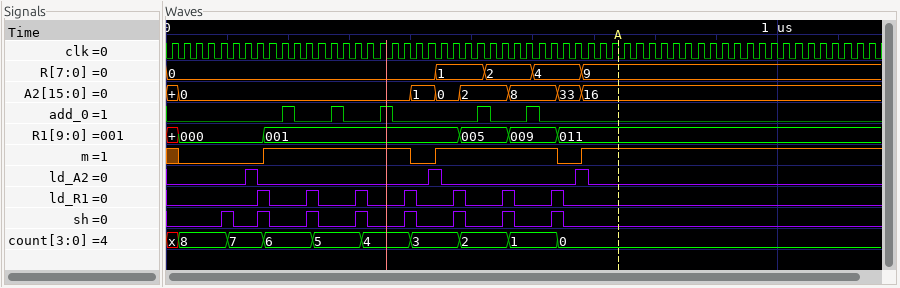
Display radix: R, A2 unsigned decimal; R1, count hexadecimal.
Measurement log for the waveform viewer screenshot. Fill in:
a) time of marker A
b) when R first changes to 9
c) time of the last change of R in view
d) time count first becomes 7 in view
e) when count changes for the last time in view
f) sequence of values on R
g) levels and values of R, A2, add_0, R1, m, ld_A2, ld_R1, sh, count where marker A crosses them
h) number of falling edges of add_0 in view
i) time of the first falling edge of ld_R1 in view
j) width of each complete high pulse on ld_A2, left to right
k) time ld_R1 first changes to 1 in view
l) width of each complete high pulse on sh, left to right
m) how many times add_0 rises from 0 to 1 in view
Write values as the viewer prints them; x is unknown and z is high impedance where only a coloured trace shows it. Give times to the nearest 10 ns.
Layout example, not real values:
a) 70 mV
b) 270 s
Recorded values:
a) 740 ns
b) 680 ns
c) 680 ns
d) 100 ns
e) 640 ns
f) 0, 1, 2, 4, 9
g) R=9, A2=16, add_0=0, R1=011, m=1, ld_A2=0, ld_R1=0, sh=0, count=0
h) 5
i) 170 ns
j) 20 ns, 20 ns, 20 ns
k) 150 ns
l) 20 ns, 20 ns, 20 ns, 20 ns, 20 ns, 20 ns, 20 ns, 20 ns
m) 5
